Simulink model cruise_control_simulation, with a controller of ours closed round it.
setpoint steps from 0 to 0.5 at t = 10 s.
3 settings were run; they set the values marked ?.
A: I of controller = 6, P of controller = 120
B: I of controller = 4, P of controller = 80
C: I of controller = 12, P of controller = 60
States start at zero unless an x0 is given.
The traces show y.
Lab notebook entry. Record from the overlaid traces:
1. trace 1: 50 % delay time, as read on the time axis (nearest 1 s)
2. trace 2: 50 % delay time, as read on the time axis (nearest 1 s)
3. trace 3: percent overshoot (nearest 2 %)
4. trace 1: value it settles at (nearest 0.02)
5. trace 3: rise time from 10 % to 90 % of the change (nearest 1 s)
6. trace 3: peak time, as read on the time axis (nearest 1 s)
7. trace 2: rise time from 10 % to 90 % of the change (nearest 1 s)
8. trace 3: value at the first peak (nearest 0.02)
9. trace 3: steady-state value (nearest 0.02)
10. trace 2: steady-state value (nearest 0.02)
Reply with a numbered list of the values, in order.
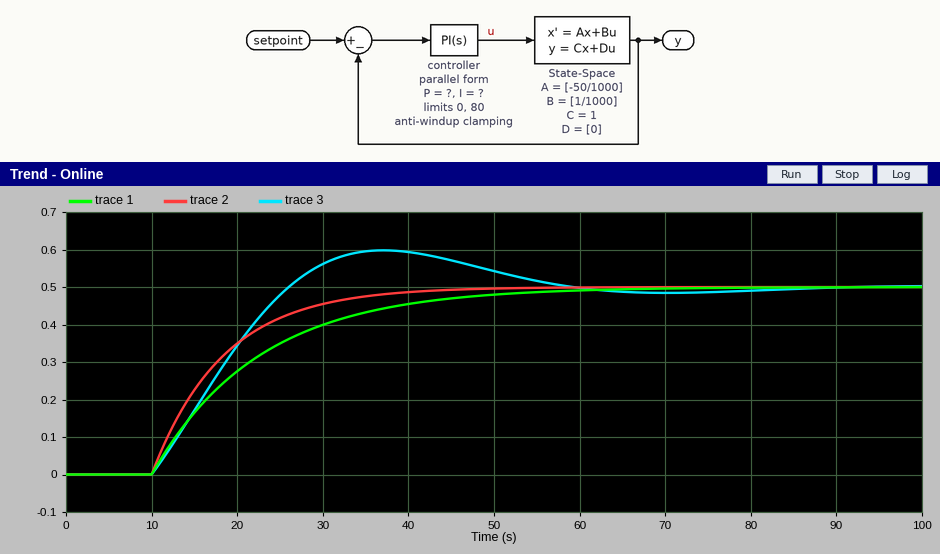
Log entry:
1. 19 s
2. 16 s
3. 20 %
4. 0.50
5. 12 s
6. 37 s
7. 18 s
8. 0.60
9. 0.50
10. 0.50
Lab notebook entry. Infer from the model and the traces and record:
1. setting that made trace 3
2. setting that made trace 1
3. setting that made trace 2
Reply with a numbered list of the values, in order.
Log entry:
1. C
2. B
3. A
